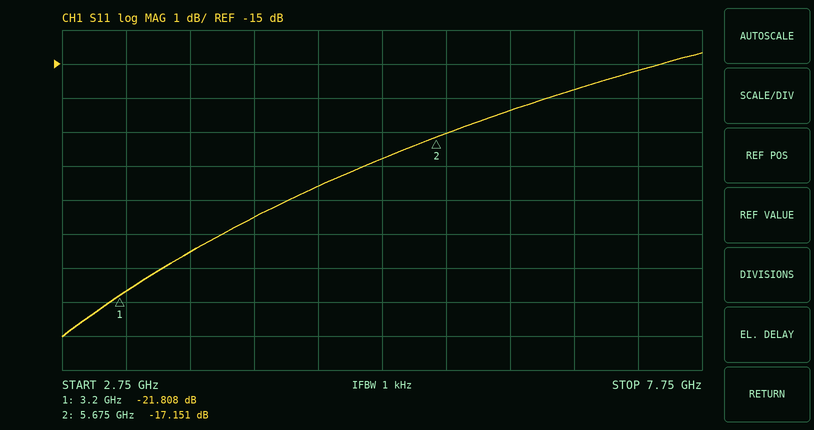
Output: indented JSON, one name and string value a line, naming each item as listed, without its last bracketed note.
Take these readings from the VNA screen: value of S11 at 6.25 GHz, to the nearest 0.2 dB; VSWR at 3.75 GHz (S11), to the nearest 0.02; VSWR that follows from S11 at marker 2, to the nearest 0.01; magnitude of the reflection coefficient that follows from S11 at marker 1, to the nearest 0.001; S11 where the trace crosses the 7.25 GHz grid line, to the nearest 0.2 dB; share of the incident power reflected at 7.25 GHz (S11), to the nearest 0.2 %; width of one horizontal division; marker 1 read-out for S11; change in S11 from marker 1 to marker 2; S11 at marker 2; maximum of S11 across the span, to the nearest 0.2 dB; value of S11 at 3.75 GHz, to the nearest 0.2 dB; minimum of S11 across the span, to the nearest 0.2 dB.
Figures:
{
  "value of S11 at 6.25 GHz, to the nearest 0.2 dB": "-16.4 dB",
  "VSWR at 3.75 GHz (S11), to the nearest 0.02": "1.20",
  "VSWR that follows from S11 at marker 2, to the nearest 0.01": "1.32",
  "magnitude of the reflection coefficient that follows from S11 at marker 1, to the nearest 0.001": "0.081",
  "S11 where the trace crosses the 7.25 GHz grid line, to the nearest 0.2 dB": "-15.2 dB",
  "share of the incident power reflected at 7.25 GHz (S11), to the nearest 0.2 %": "3.0 %",
  "width of one horizontal division": "500 MHz",
  "marker 1 read-out for S11": "-21.808 dB",
  "change in S11 from marker 1 to marker 2": "4.657 dB",
  "S11 at marker 2": "-17.151 dB",
  "maximum of S11 across the span, to the nearest 0.2 dB": "-14.6 dB",
  "value of S11 at 3.75 GHz, to the nearest 0.2 dB": "-20.6 dB",
  "minimum of S11 across the span, to the nearest 0.2 dB": "-23.0 dB"
}
